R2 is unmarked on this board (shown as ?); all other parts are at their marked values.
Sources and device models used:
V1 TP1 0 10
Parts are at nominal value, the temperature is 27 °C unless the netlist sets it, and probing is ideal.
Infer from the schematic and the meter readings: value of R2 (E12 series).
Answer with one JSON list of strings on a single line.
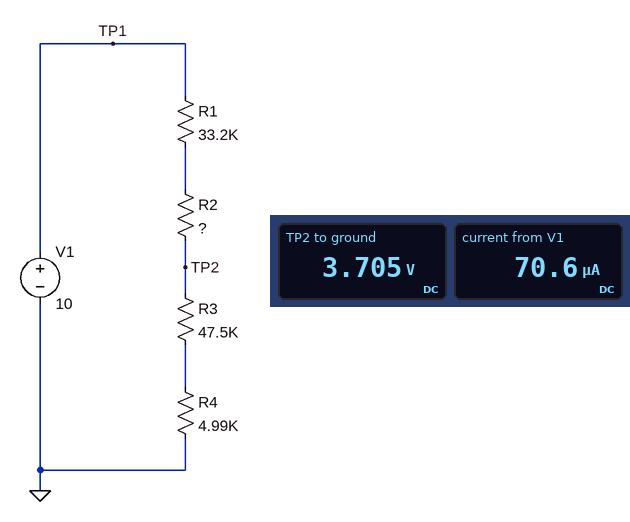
["56 kΩ"]
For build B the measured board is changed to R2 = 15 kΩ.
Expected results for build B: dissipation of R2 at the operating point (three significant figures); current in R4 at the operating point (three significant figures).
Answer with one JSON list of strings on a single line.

["148 µW", "99.3 µA"]
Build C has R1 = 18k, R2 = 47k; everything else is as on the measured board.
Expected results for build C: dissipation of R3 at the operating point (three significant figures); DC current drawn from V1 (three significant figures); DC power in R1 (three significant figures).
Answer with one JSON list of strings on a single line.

["344 µW", "85.1 µA", "130 µW"]
